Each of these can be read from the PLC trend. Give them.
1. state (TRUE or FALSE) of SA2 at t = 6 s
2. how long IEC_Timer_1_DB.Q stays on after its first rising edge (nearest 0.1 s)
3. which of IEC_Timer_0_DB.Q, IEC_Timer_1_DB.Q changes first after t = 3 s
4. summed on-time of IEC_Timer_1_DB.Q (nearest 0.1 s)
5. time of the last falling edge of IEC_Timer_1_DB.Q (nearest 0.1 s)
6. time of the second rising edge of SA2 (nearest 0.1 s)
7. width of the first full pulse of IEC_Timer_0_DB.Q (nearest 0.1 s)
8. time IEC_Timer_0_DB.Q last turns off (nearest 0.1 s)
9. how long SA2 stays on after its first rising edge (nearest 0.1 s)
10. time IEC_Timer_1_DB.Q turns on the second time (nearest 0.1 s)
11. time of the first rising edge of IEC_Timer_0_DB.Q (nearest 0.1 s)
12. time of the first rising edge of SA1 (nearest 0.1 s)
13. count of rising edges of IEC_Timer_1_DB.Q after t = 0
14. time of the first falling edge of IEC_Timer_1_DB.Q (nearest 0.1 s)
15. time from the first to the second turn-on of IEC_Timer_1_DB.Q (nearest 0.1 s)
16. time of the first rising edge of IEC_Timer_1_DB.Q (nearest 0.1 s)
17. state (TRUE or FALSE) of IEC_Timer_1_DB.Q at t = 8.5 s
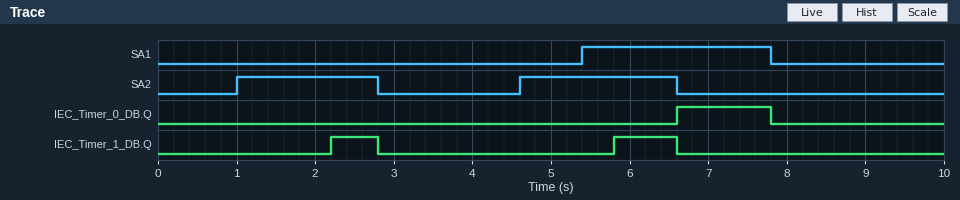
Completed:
TRUE
0.6 s
IEC_Timer_1_DB.Q
1.4 s
6.6 s
4.6 s
1.2 s
7.8 s
1.8 s
5.8 s
6.6 s
5.4 s
2
2.8 s
3.6 s
2.2 s
FALSE
